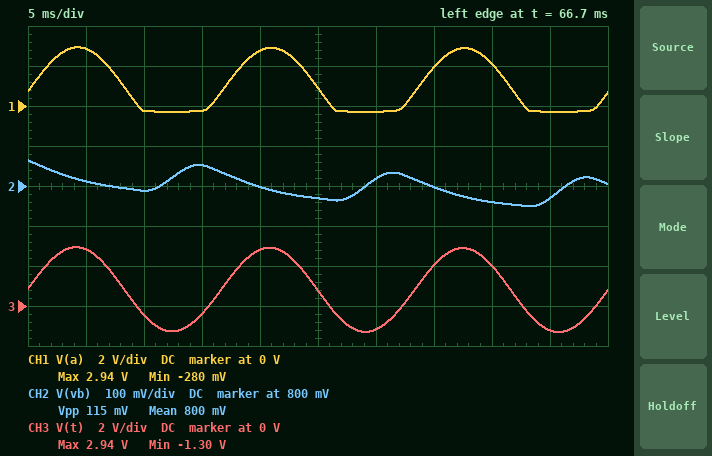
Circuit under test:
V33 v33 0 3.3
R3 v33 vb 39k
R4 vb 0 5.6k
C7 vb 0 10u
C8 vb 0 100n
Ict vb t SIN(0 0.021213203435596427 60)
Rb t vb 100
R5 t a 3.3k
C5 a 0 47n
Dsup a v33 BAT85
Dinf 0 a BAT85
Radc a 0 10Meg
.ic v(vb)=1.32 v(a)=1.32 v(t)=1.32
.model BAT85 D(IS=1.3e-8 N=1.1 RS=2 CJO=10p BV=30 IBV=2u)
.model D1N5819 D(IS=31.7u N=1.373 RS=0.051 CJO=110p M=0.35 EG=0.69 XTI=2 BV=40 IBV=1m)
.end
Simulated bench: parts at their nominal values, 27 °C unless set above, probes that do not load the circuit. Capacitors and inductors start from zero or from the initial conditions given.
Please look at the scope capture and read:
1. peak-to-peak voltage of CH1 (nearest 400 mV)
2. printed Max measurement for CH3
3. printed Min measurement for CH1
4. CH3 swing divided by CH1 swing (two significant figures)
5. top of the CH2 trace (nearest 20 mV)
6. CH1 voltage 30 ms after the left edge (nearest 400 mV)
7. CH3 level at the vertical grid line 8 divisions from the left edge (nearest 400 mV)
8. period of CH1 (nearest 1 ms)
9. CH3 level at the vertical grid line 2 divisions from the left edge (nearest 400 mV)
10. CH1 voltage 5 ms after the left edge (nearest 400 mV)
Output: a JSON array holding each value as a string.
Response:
["3.2 V", "2.94 V", "-280 mV", "1.3", "860 mV", "-400 mV", "2.0 V", "17 ms", "-400 mV", "2.8 V"]
